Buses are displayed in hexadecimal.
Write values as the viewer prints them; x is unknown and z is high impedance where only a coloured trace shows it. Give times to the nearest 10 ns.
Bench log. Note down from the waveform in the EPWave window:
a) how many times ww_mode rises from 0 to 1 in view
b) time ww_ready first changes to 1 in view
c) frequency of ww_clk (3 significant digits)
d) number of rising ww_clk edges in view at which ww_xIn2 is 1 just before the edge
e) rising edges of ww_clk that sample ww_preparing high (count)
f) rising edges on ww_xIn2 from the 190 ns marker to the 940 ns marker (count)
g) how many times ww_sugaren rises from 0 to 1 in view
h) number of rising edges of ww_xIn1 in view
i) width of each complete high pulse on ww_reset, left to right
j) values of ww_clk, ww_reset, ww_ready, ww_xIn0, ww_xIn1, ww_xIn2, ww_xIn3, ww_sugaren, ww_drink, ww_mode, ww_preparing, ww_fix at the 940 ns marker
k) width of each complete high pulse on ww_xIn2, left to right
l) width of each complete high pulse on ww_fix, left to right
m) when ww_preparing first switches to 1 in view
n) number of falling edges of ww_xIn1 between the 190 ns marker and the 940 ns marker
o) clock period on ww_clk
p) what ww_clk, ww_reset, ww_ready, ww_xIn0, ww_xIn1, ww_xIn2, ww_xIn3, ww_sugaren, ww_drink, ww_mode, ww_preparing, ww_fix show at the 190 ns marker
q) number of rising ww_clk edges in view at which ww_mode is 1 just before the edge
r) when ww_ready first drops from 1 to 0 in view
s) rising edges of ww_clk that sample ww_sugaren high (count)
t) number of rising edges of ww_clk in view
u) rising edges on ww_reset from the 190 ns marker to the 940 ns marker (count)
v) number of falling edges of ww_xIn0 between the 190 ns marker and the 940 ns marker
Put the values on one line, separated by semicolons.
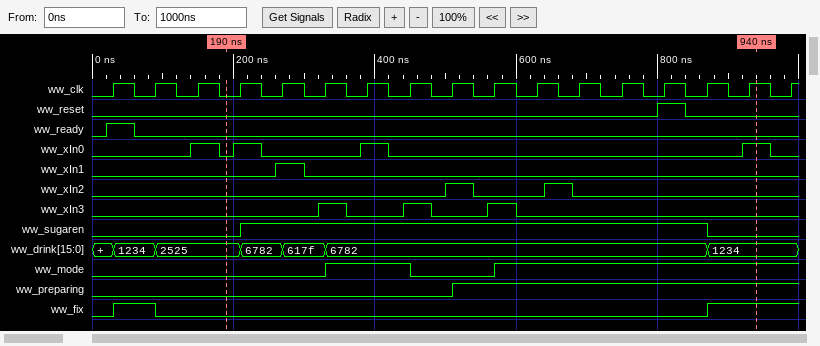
2; 20 ns; 16.7 MHz; 1; 8; 2; 1; 1; 40 ns; ww_clk=1, ww_reset=0, ww_ready=0, ww_xIn0=1, ww_xIn1=0, ww_xIn2=0, ww_xIn3=0, ww_sugaren=0, ww_drink=1234, ww_mode=1, ww_preparing=1, ww_fix=1; 40 ns, 40 ns; 60 ns; 510 ns; 1; 60 ns; ww_clk=0, ww_reset=0, ww_ready=0, ww_xIn0=0, ww_xIn1=0, ww_xIn2=0, ww_xIn3=0, ww_sugaren=0, ww_drink=2525, ww_mode=0, ww_preparing=0, ww_fix=0; 9; 60 ns; 11; 17; 1; 2
